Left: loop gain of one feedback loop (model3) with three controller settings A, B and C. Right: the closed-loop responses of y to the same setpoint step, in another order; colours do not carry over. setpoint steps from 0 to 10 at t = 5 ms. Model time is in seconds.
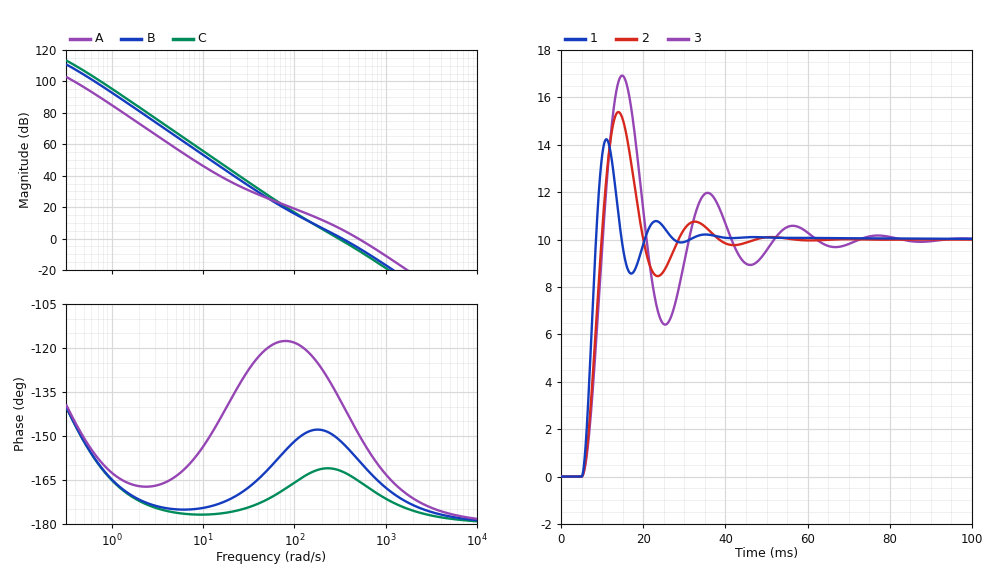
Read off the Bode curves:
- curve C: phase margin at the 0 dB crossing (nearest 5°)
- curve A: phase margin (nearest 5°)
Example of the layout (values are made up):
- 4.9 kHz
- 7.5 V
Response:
- 20°
- 30°
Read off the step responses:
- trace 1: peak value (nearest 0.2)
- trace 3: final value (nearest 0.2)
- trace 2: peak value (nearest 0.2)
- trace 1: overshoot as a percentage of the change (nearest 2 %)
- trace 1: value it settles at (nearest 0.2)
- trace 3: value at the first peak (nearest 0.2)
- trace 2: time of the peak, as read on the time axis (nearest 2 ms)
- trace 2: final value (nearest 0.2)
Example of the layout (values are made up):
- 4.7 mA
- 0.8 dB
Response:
- 14.2
- 10.0
- 15.4
- 42 %
- 10.0
- 17.0
- 14 ms
- 10.0
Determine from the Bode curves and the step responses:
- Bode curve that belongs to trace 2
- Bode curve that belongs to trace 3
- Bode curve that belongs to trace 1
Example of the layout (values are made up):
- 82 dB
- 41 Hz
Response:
- B
- C
- A
